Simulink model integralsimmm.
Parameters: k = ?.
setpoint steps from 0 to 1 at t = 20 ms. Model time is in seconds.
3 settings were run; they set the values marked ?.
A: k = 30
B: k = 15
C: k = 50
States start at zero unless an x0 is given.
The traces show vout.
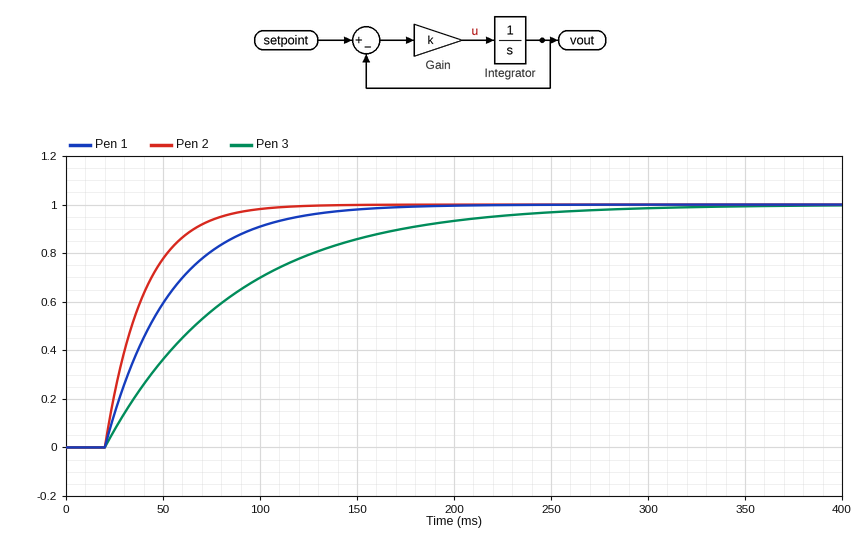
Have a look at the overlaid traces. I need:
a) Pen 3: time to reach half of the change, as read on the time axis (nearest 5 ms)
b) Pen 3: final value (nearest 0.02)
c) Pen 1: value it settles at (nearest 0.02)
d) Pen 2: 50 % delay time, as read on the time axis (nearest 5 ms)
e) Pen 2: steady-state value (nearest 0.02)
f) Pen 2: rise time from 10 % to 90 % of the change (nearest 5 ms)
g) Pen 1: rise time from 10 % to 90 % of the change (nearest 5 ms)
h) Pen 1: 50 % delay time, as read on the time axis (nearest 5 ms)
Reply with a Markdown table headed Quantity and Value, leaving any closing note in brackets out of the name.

| Quantity | Value |
|---|---|
| Pen 3: time to reach half of the change, as read on the time axis | 65 ms |
| Pen 3: final value | 1.00 |
| Pen 1: value it settles at | 1.00 |
| Pen 2: 50 % delay time, as read on the time axis | 35 ms |
| Pen 2: steady-state value | 1.00 |
| Pen 2: rise time from 10 % to 90 % of the change | 45 ms |
| Pen 1: rise time from 10 % to 90 % of the change | 75 ms |
| Pen 1: 50 % delay time, as read on the time axis | 45 ms |
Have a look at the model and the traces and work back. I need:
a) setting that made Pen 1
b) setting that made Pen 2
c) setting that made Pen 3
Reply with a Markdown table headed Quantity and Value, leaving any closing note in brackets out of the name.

| Quantity | Value |
|---|---|
| setting that made Pen 1 | A |
| setting that made Pen 2 | C |
| setting that made Pen 3 | B |
